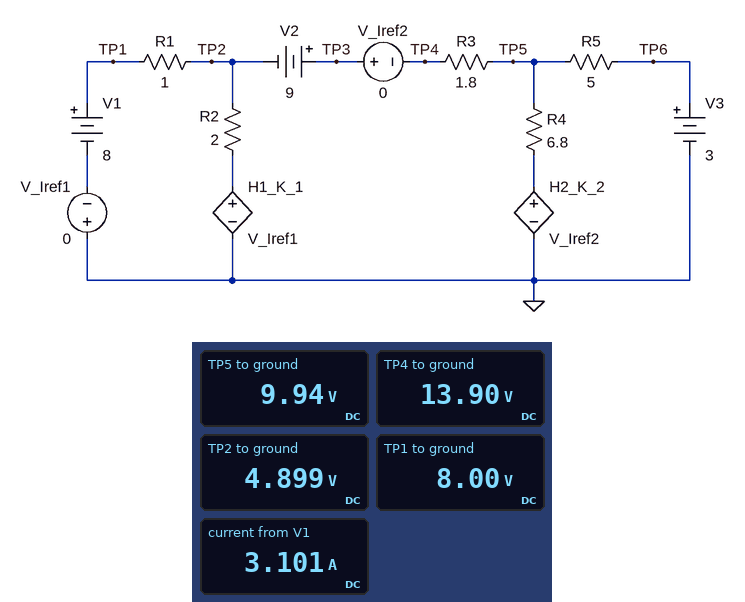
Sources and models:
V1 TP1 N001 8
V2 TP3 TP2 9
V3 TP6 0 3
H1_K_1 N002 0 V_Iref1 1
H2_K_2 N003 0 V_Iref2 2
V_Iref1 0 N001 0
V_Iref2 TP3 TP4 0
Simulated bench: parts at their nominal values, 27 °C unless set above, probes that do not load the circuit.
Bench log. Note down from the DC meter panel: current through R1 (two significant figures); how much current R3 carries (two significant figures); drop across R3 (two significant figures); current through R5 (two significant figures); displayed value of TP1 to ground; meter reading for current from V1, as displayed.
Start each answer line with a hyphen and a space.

- 3.1 A
- 2.2 A
- 4.0 V
- 1.4 A
- 8.00 V
- 3.101 A
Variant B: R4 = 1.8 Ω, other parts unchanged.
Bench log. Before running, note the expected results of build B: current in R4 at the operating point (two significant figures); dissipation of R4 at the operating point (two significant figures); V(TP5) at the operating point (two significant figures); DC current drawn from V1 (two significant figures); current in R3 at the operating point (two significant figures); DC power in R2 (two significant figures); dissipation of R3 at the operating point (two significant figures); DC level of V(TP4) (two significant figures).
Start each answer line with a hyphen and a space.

- 1.7 A
- 5.0 W
- 8.6 V
- 3.4 A
- 2.8 A
- 730 mW
- 14 W
- 14 V
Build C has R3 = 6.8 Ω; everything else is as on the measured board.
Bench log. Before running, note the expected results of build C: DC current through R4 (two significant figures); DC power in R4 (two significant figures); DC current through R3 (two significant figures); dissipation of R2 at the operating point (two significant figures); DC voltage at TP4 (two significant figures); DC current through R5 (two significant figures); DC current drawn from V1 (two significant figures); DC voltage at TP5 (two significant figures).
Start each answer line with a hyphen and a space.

- 560 mA
- 2.1 W
- 1.2 A
- 3.9 W
- 14 V
- 640 mA
- 2.6 A
- 6.2 V
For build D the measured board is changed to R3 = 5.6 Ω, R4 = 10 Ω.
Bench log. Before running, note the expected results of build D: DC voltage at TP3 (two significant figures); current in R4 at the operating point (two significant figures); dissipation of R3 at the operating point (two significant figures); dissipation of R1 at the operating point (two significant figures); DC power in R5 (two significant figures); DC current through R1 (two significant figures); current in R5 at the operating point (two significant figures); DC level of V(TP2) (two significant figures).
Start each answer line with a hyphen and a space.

- 14 V
- 460 mA
- 9.3 W
- 7.0 W
- 3.4 W
- 2.6 A
- 830 mA
- 5.4 V
